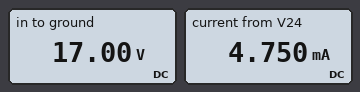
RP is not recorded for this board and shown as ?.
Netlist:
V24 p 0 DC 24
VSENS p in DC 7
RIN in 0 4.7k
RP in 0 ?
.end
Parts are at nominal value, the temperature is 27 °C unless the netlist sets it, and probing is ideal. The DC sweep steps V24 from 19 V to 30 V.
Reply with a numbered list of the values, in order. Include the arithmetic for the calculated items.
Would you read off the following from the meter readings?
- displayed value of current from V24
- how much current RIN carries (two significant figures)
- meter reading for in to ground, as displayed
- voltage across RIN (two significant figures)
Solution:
1. 4.750 mA
2. (17 V) / 4.7 kΩ = 3.6 mA
3. 17.00 V
4. 17 V = 17 V
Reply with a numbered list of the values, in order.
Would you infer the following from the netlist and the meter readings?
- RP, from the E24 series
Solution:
1. 15 kΩ
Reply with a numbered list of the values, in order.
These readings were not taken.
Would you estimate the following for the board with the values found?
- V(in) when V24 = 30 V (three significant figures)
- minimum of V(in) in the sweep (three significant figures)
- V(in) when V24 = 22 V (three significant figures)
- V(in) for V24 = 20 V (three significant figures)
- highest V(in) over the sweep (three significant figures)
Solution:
1. 23.0 V
2. 12.0 V
3. 15.0 V
4. 13.0 V
5. 23.0 V
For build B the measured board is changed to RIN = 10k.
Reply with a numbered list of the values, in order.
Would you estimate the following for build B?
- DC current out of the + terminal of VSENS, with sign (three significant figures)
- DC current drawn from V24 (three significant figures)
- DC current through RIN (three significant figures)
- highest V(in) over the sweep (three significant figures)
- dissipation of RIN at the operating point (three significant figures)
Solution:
1. -2.83 mA
2. 2.83 mA
3. 1.70 mA
4. 23.0 V
5. 28.9 mW
